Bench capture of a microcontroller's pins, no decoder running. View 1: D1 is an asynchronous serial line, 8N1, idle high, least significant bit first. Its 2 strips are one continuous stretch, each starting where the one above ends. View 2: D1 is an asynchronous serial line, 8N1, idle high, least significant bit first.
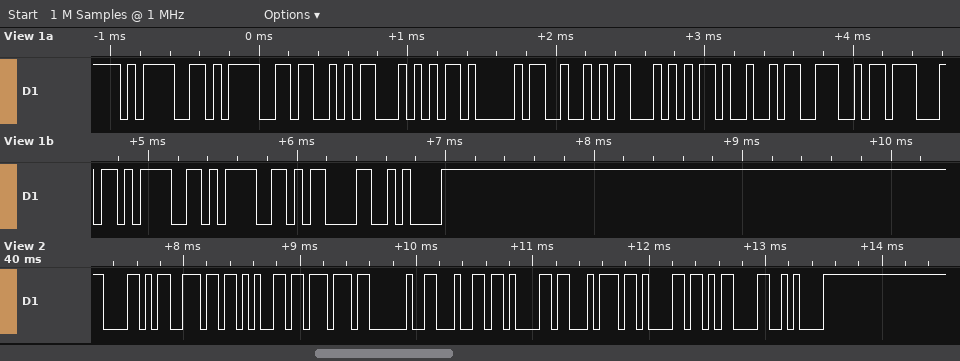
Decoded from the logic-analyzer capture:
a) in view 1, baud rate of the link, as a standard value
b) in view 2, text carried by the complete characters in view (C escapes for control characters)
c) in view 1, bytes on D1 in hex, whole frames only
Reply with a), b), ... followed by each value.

a) 19200 baud
b) "Xnew data\r\n"
c) 0x3D 0x3D 0x53 0x54 0x41 0x52 0x54 0x49 0x4E 0x47 0x3D 0x3D 0x0D 0x0A
